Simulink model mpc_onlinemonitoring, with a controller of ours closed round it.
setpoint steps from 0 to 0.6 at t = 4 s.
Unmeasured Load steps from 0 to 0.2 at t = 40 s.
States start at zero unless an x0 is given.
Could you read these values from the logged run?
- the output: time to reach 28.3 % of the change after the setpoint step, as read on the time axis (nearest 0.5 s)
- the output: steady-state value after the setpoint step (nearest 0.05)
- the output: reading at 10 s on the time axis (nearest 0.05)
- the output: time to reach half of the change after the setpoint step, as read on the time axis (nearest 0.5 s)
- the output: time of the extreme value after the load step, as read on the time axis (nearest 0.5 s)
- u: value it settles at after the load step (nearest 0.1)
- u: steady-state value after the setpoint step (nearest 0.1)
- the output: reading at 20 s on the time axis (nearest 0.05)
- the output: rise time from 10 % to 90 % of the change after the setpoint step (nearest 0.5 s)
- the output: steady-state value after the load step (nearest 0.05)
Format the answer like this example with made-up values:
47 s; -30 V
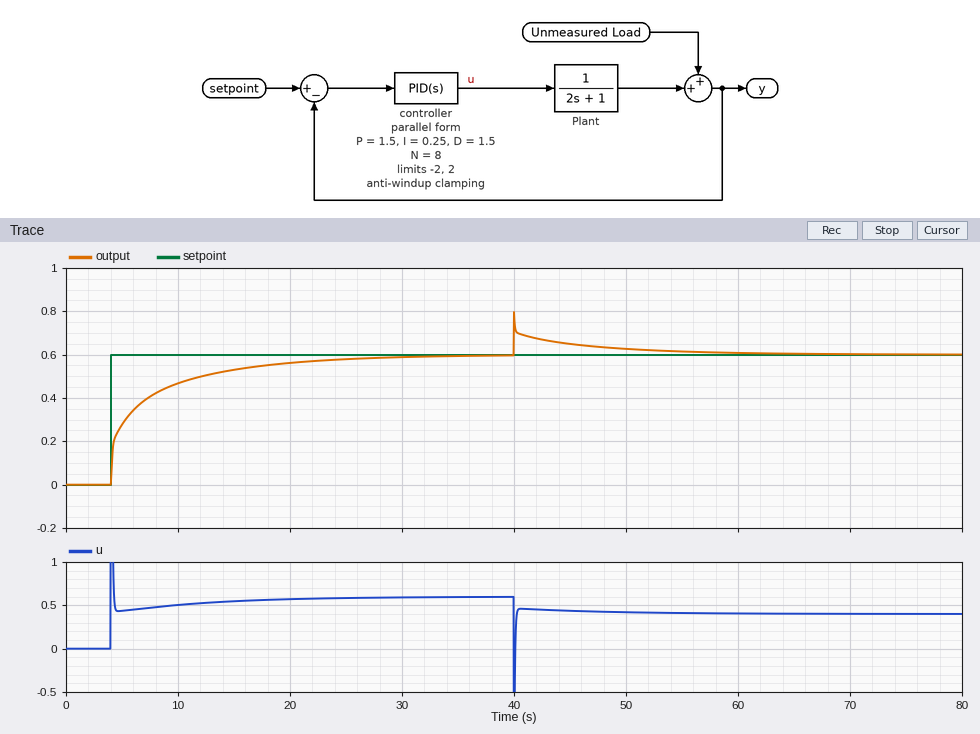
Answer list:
4.0 s; 0.60; 0.45; 5.5 s; 40.0 s; 0.4; 0.6; 0.55; 12.0 s; 0.60
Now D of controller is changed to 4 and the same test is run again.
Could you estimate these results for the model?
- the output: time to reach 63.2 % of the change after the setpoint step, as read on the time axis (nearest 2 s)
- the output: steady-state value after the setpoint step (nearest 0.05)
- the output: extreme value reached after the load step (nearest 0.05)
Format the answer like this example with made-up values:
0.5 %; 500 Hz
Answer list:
8 s; 0.60; 0.80
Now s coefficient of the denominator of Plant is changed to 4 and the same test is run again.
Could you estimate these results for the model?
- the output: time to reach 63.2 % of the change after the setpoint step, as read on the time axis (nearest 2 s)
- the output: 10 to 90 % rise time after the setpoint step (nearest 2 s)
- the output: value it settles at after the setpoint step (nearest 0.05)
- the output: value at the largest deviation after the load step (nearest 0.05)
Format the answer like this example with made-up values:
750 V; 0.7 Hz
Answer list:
8 s; 10 s; 0.60; 0.80
